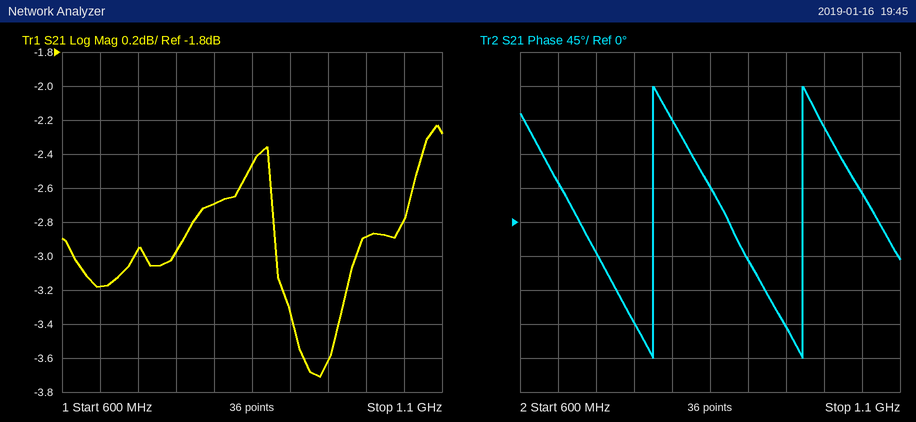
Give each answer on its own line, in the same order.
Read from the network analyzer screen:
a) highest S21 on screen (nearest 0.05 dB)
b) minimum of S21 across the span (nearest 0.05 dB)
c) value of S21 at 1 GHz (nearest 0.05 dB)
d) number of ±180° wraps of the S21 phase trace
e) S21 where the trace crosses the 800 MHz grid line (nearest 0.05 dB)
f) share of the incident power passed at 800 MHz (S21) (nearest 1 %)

-2.25 dB
-3.70 dB
-2.90 dB
2
-2.70 dB
54 %
